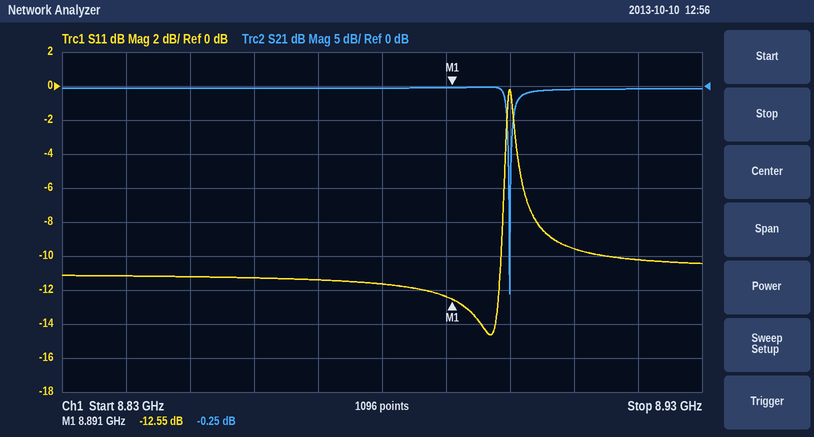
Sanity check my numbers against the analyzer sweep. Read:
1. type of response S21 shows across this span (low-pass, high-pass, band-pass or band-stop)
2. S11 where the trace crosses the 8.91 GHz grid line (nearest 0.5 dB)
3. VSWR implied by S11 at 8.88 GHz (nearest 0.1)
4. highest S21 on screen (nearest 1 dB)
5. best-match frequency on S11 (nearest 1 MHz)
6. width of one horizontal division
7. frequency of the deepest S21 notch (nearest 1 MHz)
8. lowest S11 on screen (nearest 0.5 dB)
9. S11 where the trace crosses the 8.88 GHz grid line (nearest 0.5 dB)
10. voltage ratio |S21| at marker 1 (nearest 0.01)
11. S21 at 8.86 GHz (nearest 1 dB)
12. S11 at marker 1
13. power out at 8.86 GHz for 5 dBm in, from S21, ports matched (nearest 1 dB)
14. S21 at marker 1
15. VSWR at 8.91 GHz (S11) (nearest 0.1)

band-stop
-9.5 dB
1.7
0 dB
8.897 GHz
10 MHz
8.900 GHz
-14.5 dB
-11.5 dB
0.97
0 dB
-12.55 dB
5 dBm
-0.25 dB
2.0
